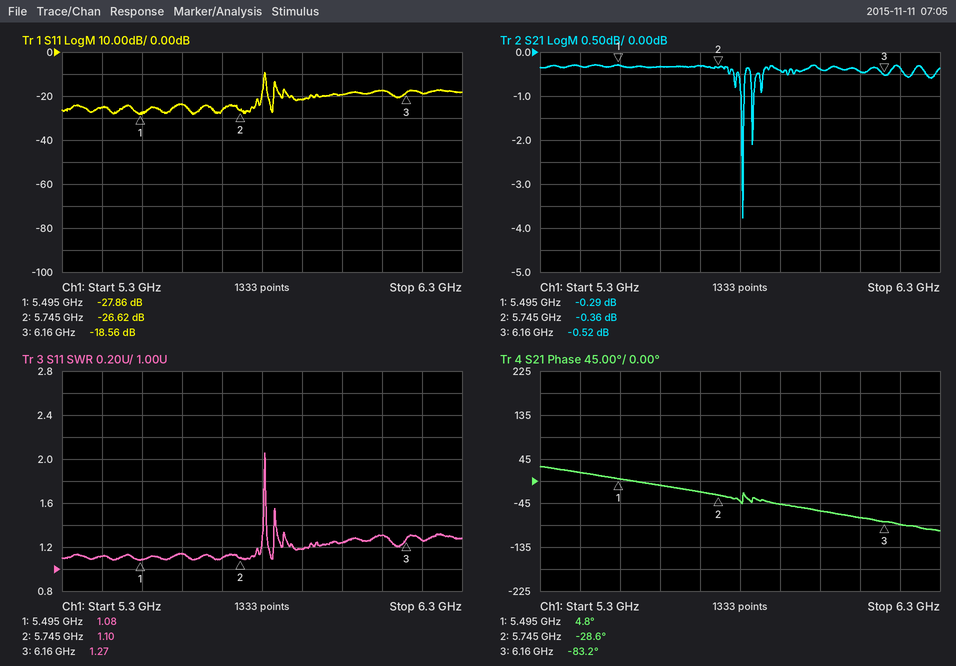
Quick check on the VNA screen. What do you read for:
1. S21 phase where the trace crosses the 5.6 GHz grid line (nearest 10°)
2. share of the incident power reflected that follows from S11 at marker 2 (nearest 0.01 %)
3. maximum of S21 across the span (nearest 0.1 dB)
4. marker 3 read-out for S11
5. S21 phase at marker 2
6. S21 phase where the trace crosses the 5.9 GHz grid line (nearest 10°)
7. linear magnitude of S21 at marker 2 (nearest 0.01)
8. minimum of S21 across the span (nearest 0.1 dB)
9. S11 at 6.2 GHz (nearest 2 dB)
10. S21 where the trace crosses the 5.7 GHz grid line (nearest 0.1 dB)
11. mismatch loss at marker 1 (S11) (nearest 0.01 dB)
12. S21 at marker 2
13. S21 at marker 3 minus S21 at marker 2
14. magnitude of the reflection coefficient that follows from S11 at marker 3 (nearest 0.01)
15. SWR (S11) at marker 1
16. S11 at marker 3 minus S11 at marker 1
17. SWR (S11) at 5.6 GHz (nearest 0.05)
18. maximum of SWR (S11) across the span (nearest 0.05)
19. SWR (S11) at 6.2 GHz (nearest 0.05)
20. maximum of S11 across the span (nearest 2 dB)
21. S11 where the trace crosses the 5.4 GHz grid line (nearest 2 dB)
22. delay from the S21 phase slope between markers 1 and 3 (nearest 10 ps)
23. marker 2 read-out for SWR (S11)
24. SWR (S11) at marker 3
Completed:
-10°
0.22 %
-0.3 dB
-18.56 dB
-28.6°
-50°
0.96
-3.8 dB
-18 dB
-0.3 dB
0.01 dB
-0.36 dB
-0.16 dB
0.12
1.08
9.30 dB
1.15
2.05
1.25
-10 dB
-26 dB
370 ps
1.10
1.27
